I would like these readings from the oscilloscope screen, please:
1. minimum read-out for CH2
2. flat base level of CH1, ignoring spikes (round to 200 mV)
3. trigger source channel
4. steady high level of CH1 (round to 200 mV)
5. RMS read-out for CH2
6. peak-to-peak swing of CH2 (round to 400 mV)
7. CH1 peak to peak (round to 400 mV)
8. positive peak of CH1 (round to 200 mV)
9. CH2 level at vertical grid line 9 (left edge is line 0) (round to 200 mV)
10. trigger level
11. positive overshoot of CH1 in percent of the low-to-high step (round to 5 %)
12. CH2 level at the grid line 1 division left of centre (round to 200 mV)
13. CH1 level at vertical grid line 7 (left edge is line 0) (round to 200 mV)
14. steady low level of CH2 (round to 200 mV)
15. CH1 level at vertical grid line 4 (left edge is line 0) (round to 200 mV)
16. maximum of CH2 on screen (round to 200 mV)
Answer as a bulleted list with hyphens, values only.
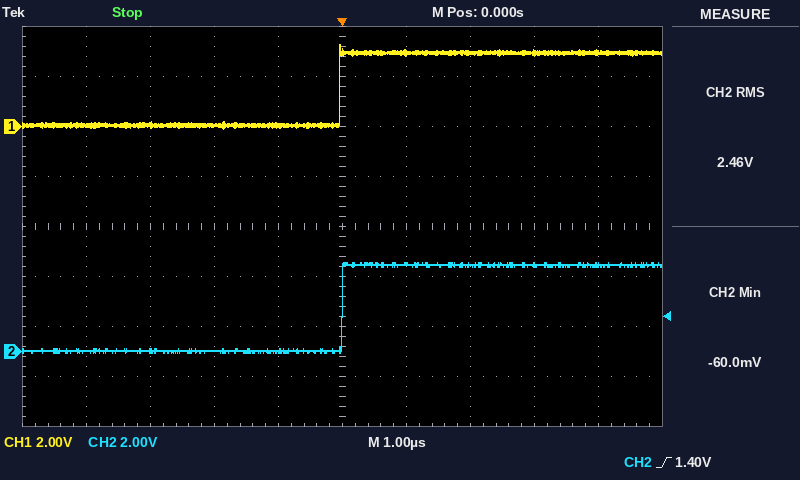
- -60.0 mV
- 0.0 V
- CH2
- 3.0 V
- 2.46 V
- 3.6 V
- 3.2 V
- 3.2 V
- 3.4 V
- 1.40 V
- 10 %
- 0.0 V
- 3.0 V
- 0.0 V
- 0.0 V
- 3.6 V
